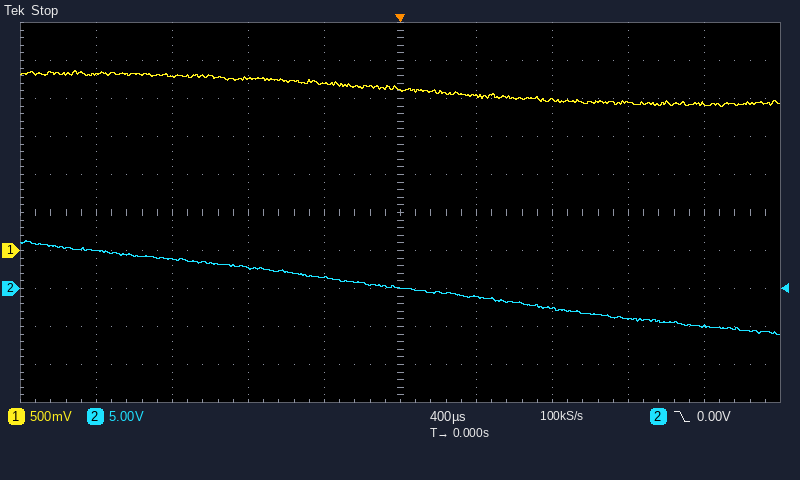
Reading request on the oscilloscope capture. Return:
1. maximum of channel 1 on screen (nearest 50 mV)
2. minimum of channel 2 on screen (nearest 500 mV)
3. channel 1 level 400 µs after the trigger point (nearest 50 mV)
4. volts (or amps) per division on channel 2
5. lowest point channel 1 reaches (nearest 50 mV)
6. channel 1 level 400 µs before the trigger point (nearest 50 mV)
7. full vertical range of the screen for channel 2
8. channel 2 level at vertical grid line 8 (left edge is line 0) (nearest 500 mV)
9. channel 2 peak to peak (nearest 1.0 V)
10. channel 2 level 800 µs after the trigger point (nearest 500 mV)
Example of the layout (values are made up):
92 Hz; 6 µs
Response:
2.35 V; -6.0 V; 2.05 V; 5 V; 1.90 V; 2.20 V; 50 V; -4.0 V; 12.0 V; -2.5 V
